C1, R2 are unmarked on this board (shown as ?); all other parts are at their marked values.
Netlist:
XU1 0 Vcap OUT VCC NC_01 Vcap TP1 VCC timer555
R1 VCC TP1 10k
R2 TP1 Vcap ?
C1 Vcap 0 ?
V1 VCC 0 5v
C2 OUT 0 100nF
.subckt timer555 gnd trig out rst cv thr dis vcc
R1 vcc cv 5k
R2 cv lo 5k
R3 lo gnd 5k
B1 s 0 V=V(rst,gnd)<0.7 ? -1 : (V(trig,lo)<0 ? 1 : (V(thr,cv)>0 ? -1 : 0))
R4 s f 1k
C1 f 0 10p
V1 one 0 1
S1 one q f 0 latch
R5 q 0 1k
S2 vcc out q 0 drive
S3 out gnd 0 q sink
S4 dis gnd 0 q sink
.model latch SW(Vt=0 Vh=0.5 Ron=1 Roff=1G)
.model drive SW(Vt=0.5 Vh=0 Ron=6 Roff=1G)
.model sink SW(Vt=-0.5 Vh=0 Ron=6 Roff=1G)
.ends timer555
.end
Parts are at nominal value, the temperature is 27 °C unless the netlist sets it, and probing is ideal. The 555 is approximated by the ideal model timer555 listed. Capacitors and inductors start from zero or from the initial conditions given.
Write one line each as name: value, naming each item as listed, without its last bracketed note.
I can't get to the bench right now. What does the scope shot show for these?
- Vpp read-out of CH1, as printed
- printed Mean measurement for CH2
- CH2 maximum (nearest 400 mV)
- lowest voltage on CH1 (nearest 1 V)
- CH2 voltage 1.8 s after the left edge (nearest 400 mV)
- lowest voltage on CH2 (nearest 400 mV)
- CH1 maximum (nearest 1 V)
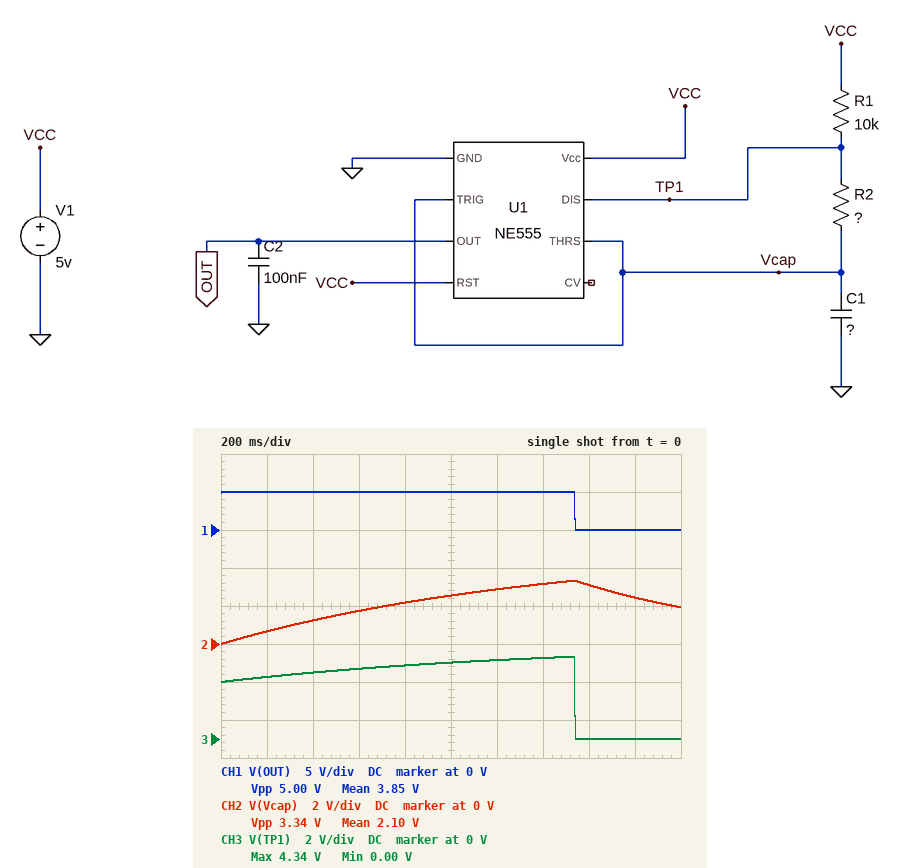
Vpp read-out of CH1, as printed: 5.00 V
printed Mean measurement for CH2: 2.10 V
CH2 maximum: 3.2 V
lowest voltage on CH1: 0 V
CH2 voltage 1.8 s after the left edge: 2.4 V
lowest voltage on CH2: 0 V
CH1 maximum: 5 V
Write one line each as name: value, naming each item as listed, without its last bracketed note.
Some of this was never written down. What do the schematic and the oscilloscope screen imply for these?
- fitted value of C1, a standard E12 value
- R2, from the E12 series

fitted value of C1, a standard E12 value: 56 µF
R2, from the E12 series: 15 kΩ
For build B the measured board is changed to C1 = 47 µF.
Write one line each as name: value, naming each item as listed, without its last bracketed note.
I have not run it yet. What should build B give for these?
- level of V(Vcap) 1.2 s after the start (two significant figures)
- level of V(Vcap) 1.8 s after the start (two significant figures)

level of V(Vcap) 1.2 s after the start: 3.2 V
level of V(Vcap) 1.8 s after the start: 1.7 V
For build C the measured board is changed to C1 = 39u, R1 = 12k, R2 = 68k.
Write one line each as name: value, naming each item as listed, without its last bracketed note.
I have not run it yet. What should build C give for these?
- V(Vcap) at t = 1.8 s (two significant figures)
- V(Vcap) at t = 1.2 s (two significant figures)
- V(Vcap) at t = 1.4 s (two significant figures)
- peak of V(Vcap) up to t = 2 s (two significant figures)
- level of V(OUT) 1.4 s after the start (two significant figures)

V(Vcap) at t = 1.8 s: 2.2 V
V(Vcap) at t = 1.2 s: 1.6 V
V(Vcap) at t = 1.4 s: 1.8 V
peak of V(Vcap) up to t = 2 s: 2.4 V
level of V(OUT) 1.4 s after the start: 5.0 V
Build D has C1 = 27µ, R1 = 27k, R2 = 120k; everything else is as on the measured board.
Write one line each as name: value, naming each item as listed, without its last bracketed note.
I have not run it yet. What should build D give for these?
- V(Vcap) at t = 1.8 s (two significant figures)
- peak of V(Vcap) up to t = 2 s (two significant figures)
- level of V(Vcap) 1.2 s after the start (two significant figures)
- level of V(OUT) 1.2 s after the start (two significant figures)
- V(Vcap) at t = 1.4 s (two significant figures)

V(Vcap) at t = 1.8 s: 1.8 V
peak of V(Vcap) up to t = 2 s: 2.0 V
level of V(Vcap) 1.2 s after the start: 1.3 V
level of V(OUT) 1.2 s after the start: 5.0 V
V(Vcap) at t = 1.4 s: 1.5 V
